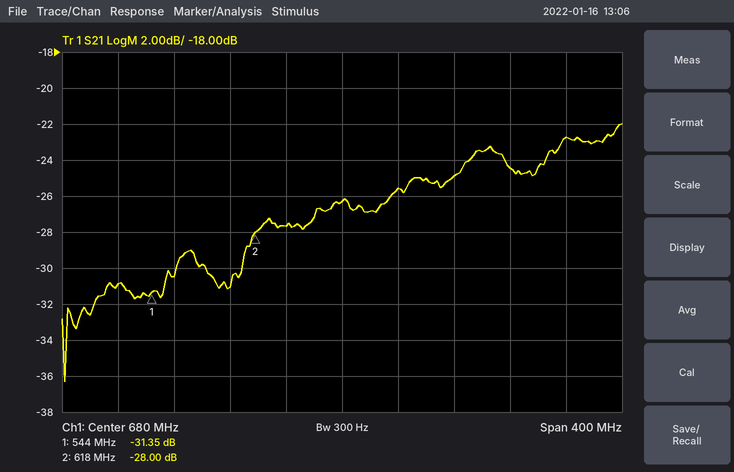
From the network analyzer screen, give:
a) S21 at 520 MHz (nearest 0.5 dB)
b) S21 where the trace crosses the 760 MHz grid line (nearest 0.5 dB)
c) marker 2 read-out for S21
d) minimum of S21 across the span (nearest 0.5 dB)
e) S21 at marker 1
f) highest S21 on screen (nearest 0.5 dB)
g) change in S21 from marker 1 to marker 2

-31.0 dB
-25.0 dB
-28.00 dB
-36.5 dB
-31.35 dB
-22.0 dB
3.35 dB
